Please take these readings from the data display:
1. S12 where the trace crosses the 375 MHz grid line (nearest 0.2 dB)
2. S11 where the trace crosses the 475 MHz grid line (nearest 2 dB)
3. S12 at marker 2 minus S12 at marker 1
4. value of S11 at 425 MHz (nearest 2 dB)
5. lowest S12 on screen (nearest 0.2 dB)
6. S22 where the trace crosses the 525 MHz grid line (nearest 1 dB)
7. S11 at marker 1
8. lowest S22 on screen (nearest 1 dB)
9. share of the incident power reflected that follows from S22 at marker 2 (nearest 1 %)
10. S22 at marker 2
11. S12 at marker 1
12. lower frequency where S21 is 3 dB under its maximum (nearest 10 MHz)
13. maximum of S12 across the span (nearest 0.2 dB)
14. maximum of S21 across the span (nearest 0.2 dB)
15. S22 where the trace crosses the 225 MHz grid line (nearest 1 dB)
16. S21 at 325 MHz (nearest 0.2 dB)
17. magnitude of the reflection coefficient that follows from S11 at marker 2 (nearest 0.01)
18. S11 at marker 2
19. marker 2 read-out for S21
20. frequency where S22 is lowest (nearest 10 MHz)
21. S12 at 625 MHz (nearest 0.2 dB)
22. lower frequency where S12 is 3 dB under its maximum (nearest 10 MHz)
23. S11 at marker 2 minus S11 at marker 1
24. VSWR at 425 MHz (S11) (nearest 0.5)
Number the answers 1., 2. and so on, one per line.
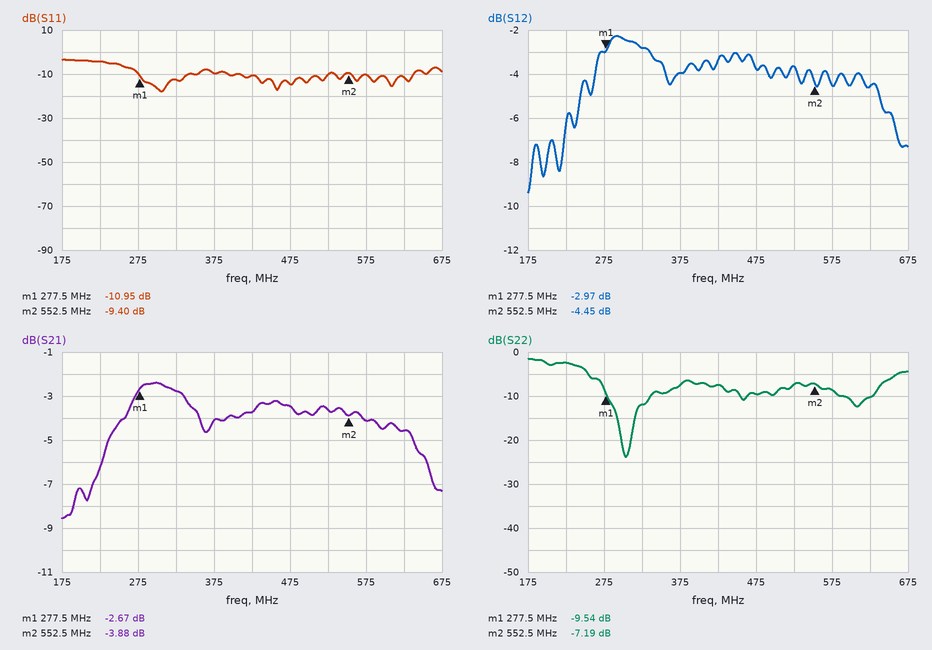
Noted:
1. -4.0 dB
2. -14 dB
3. -1.48 dB
4. -10 dB
5. -9.4 dB
6. -7 dB
7. -10.95 dB
8. -24 dB
9. 19 %
10. -7.19 dB
11. -2.97 dB
12. 230 MHz
13. -2.2 dB
14. -2.4 dB
15. -2 dB
16. -2.8 dB
17. 0.34
18. -9.40 dB
19. -3.88 dB
20. 300 MHz
21. -4.6 dB
22. 240 MHz
23. 1.55 dB
24. 2.0
